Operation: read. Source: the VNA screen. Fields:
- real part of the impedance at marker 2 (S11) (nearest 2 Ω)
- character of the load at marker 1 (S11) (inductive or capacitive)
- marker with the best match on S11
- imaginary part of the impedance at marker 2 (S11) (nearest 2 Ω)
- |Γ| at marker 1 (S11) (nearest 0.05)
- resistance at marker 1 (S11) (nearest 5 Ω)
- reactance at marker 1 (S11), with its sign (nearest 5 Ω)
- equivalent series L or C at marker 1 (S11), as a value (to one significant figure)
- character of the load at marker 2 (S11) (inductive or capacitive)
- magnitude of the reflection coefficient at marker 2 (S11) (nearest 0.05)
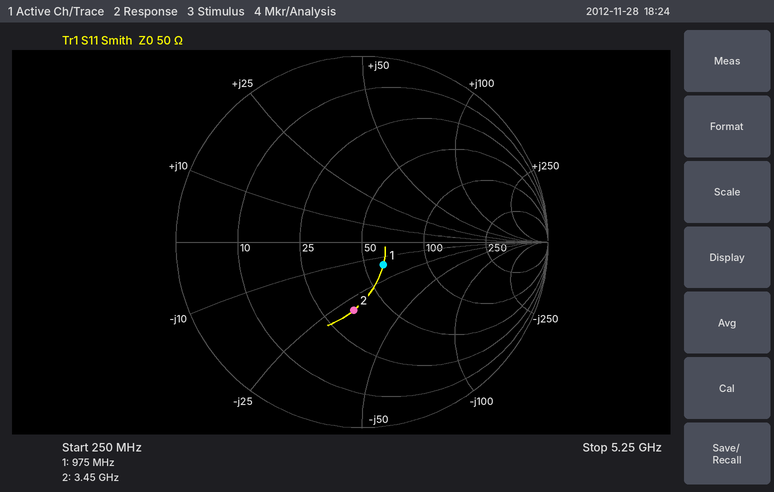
36 Ω
capacitive
marker 1
-30 Ω
0.15
60 Ω
-15 Ω
10 pF
capacitive
0.35
